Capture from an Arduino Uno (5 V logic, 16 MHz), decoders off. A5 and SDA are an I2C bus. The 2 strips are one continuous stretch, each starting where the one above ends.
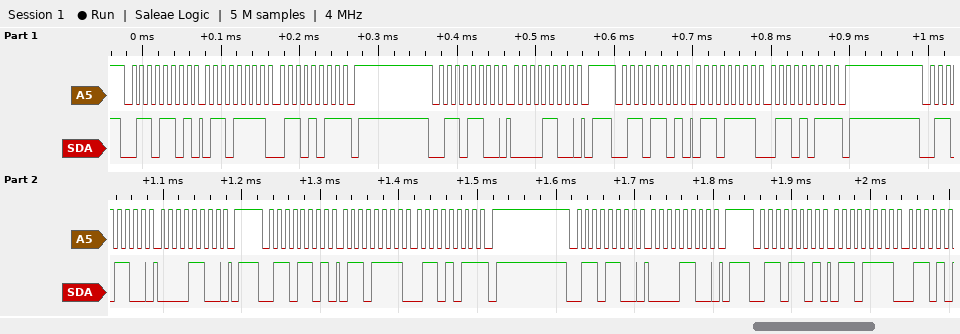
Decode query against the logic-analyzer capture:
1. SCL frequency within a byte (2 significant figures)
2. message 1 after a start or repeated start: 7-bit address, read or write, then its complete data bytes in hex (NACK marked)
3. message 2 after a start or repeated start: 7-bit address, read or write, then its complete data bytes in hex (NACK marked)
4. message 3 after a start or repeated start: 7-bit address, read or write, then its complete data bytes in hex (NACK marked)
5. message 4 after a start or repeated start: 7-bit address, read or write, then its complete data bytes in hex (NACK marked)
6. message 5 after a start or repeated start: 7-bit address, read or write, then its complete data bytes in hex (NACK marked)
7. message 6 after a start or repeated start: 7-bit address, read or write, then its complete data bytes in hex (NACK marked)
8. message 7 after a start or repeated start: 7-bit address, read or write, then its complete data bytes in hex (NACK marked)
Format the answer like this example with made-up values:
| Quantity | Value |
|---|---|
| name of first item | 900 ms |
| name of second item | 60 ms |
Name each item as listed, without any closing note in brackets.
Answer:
| Quantity | Value |
|---|---|
| SCL frequency within a byte | 100 kHz |
| message 1 after a start or repeated start: 7-bit address, read or write, then its complete data bytes in hex | 0x36 read: 6F 6B NACK |
| message 2 after a start or repeated start: 7-bit address, read or write, then its complete data bytes in hex | 0x36 write: 0C |
| message 3 after a start or repeated start: 7-bit address, read or write, then its complete data bytes in hex | 0x36 read: 6F 6B NACK |
| message 4 after a start or repeated start: 7-bit address, read or write, then its complete data bytes in hex | 0x36 write: 0C |
| message 5 after a start or repeated start: 7-bit address, read or write, then its complete data bytes in hex | 0x36 read: 6F 6B NACK |
| message 6 after a start or repeated start: 7-bit address, read or write, then its complete data bytes in hex | 0x36 write: 0C |
| message 7 after a start or repeated start: 7-bit address, read or write, then its complete data bytes in hex | 0x36 read: 6F |
